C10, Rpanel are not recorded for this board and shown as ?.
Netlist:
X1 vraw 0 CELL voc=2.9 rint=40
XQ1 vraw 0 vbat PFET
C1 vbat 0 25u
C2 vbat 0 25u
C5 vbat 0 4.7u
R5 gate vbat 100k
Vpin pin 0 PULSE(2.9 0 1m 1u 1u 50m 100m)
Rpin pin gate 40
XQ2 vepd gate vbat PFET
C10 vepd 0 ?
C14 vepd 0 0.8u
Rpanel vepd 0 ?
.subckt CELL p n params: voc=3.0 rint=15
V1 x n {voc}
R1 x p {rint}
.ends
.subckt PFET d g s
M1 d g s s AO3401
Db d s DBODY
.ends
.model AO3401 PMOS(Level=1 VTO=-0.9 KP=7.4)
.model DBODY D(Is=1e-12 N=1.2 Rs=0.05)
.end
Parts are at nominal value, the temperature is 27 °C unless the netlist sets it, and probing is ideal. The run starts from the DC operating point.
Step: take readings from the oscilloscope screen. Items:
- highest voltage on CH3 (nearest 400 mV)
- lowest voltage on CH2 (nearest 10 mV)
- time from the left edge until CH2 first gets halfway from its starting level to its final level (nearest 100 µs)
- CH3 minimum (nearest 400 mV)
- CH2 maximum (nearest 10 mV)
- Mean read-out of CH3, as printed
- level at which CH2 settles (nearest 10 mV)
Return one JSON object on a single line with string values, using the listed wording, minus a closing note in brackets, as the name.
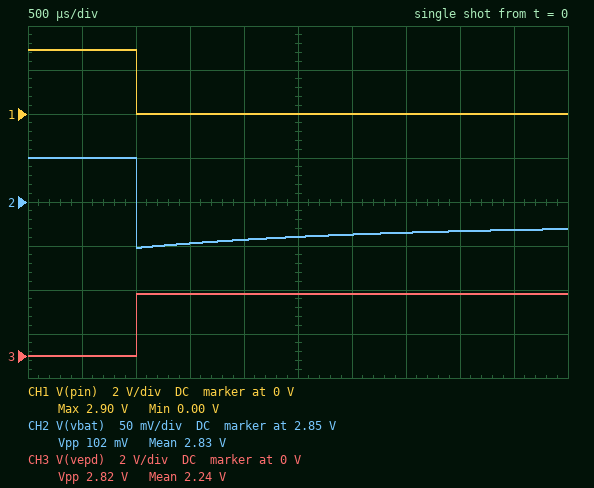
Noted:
{"highest voltage on CH3": "2.8 V", "lowest voltage on CH2": "2.80 V", "time from the left edge until CH2 first gets halfway from its starting level to its final level": "1.0 ms", "CH3 minimum": "0 V", "CH2 maximum": "2.90 V", "Mean read-out of CH3, as printed": "2.24 V", "level at which CH2 settles": "2.82 V"}
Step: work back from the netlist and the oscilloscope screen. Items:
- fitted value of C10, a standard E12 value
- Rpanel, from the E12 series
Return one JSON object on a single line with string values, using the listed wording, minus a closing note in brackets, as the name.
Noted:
{"fitted value of C10, a standard E12 value": "1.2 µF", "Rpanel, from the E12 series": "1.5 kΩ"}
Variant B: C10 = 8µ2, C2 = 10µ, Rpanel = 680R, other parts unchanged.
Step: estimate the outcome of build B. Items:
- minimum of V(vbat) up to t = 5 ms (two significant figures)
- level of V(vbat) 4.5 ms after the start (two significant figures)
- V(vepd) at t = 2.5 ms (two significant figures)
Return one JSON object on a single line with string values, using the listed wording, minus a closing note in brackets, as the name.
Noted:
{"minimum of V(vbat) up to t = 5 ms": "2.4 V", "level of V(vbat) 4.5 ms after the start": "2.7 V", "V(vepd) at t = 2.5 ms": "2.6 V"}
